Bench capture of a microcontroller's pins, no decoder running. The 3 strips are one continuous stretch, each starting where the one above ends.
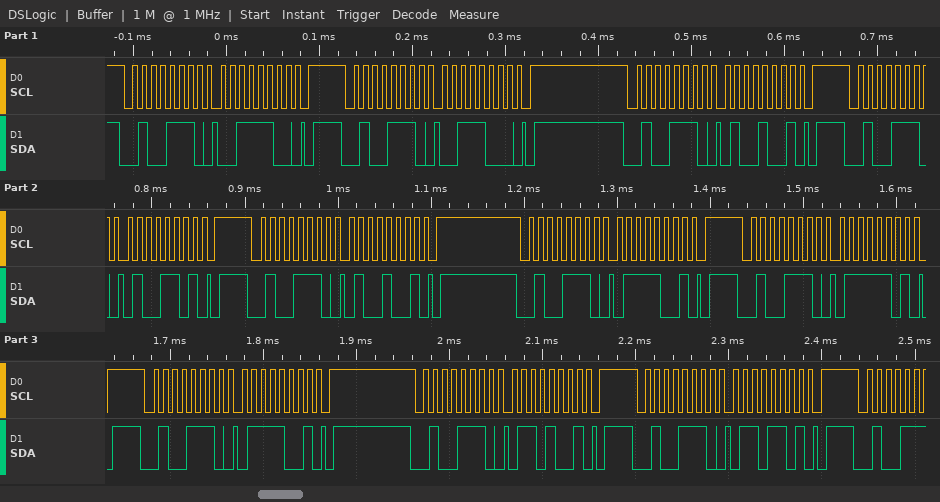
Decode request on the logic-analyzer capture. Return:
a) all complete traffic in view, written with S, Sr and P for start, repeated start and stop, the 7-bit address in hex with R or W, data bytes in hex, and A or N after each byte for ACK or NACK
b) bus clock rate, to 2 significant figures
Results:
S 27W A 3C A P S 27W A 38 A P S 27W A 49 A P S 27W A 4D A P S 27W A 49 A P S 27W A 79 A P S 27W A 7D A P S 27W A 79 A P S 27W A 69 A P S 27W A 6D A P
100 kHz
